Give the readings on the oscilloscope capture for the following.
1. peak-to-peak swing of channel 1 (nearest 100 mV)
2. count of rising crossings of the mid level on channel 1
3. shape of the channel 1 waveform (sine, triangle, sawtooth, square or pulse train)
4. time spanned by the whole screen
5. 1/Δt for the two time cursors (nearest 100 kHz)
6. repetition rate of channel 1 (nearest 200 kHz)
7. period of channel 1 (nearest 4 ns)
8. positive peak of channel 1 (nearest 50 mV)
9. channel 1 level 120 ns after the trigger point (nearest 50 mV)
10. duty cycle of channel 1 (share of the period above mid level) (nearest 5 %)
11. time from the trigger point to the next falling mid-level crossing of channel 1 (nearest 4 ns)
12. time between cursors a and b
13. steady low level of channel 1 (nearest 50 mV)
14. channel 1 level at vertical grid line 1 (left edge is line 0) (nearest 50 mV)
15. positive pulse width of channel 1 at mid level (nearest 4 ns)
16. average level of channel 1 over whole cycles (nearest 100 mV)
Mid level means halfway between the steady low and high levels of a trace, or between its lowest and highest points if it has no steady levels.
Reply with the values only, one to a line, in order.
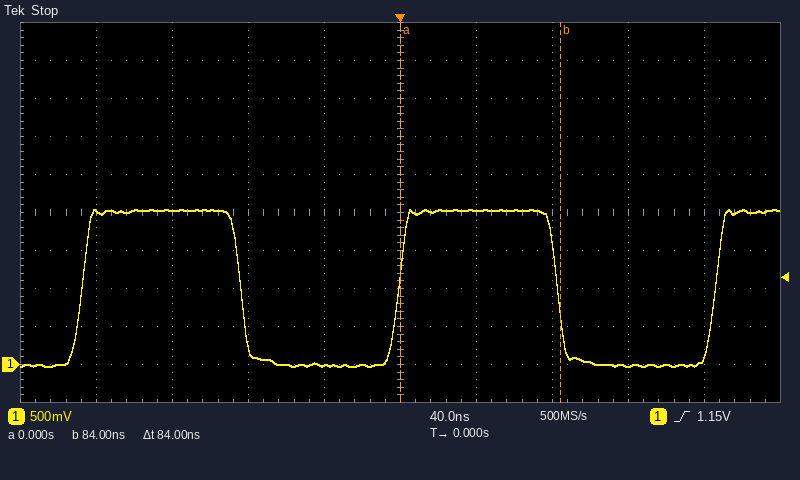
2.10 V
3
square
400 ns
11.9 MHz
6.0 MHz
168 ns
2.05 V
0 mV
50 %
84 ns
84 ns
0 mV
2.00 V
84 ns
1.0 V
